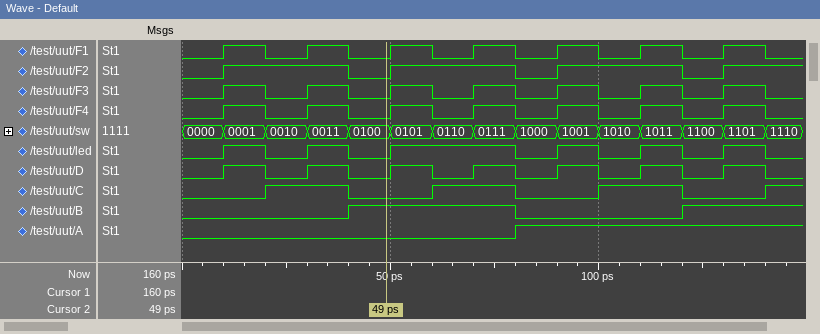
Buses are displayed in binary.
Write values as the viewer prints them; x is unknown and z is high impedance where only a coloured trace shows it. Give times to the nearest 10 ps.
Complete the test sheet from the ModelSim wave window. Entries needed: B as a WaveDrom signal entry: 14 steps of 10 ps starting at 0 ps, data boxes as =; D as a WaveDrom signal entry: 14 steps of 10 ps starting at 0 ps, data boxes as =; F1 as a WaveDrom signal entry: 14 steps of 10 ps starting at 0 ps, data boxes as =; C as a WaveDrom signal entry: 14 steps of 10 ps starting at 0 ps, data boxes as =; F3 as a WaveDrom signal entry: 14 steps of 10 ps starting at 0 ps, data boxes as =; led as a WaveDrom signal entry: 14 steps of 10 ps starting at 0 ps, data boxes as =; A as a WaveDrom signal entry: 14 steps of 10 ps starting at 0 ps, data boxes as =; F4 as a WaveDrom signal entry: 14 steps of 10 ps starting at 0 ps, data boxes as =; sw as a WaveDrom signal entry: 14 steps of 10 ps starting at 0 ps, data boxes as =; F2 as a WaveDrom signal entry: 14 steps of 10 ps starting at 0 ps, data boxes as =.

{name: 'B', wave: '0...1...0...1.'}
{name: 'D', wave: '01010101010101'}
{name: 'F1', wave: '01010101010101'}
{name: 'C', wave: '0.1.0.1.0.1.0.'}
{name: 'F3', wave: '01010101010101'}
{name: 'led', wave: '010101..010101'}
{name: 'A', wave: '0.......1.....'}
{name: 'F4', wave: '01010101010101'}
{name: 'sw', wave: '==============', data: '0000 0001 0010 0011 0100 0101 0110 0111 1000 1001 1010 1011 1100 1101'}
{name: 'F2', wave: '01..01..01..01'}
